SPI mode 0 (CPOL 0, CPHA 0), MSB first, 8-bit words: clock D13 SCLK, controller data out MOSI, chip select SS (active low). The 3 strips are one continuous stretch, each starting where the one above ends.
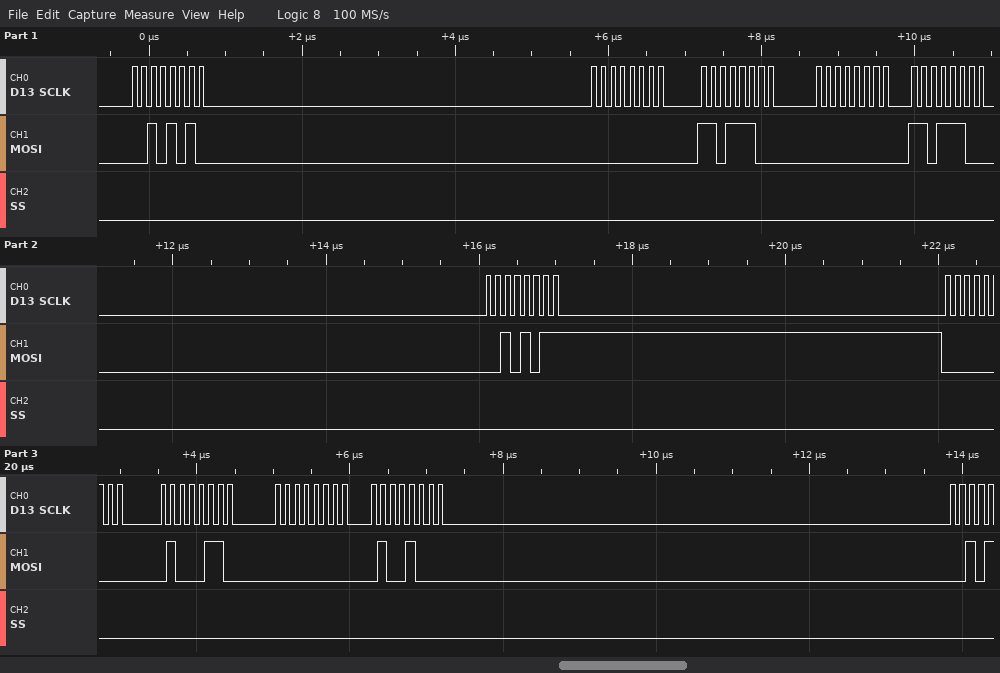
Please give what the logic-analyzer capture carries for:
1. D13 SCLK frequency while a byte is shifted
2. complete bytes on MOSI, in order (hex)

8 MHz
0x2A 0x00 0xDC 0x00 0xDC 0x2B 0x00 0x46 0x00 0x48
